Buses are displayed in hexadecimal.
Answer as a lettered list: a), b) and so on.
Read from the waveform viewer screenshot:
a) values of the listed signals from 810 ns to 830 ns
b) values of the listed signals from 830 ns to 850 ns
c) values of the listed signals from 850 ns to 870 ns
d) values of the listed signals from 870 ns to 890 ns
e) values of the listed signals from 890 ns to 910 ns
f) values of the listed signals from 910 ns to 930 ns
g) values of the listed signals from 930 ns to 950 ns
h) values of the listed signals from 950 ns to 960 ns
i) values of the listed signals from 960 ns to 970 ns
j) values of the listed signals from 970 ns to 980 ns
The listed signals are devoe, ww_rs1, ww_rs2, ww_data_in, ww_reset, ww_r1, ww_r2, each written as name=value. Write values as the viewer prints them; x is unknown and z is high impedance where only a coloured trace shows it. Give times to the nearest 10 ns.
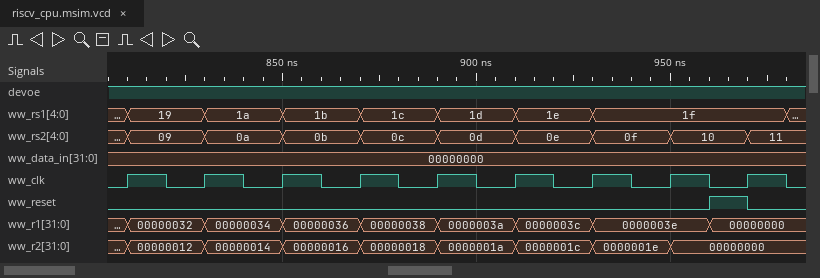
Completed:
a) devoe=1, ww_rs1=19, ww_rs2=09, ww_data_in=00000000, ww_reset=0, ww_r1=00000032, ww_r2=00000012
b) devoe=1, ww_rs1=1a, ww_rs2=0a, ww_data_in=00000000, ww_reset=0, ww_r1=00000034, ww_r2=00000014
c) devoe=1, ww_rs1=1b, ww_rs2=0b, ww_data_in=00000000, ww_reset=0, ww_r1=00000036, ww_r2=00000016
d) devoe=1, ww_rs1=1c, ww_rs2=0c, ww_data_in=00000000, ww_reset=0, ww_r1=00000038, ww_r2=00000018
e) devoe=1, ww_rs1=1d, ww_rs2=0d, ww_data_in=00000000, ww_reset=0, ww_r1=0000003a, ww_r2=0000001a
f) devoe=1, ww_rs1=1e, ww_rs2=0e, ww_data_in=00000000, ww_reset=0, ww_r1=0000003c, ww_r2=0000001c
g) devoe=1, ww_rs1=1f, ww_rs2=0f, ww_data_in=00000000, ww_reset=0, ww_r1=0000003e, ww_r2=0000001e
h) devoe=1, ww_rs1=1f, ww_rs2=10, ww_data_in=00000000, ww_reset=0, ww_r1=0000003e, ww_r2=00000000
i) devoe=1, ww_rs1=1f, ww_rs2=10, ww_data_in=00000000, ww_reset=1, ww_r1=00000000, ww_r2=00000000
j) devoe=1, ww_rs1=1f, ww_rs2=11, ww_data_in=00000000, ww_reset=0, ww_r1=00000000, ww_r2=00000000
